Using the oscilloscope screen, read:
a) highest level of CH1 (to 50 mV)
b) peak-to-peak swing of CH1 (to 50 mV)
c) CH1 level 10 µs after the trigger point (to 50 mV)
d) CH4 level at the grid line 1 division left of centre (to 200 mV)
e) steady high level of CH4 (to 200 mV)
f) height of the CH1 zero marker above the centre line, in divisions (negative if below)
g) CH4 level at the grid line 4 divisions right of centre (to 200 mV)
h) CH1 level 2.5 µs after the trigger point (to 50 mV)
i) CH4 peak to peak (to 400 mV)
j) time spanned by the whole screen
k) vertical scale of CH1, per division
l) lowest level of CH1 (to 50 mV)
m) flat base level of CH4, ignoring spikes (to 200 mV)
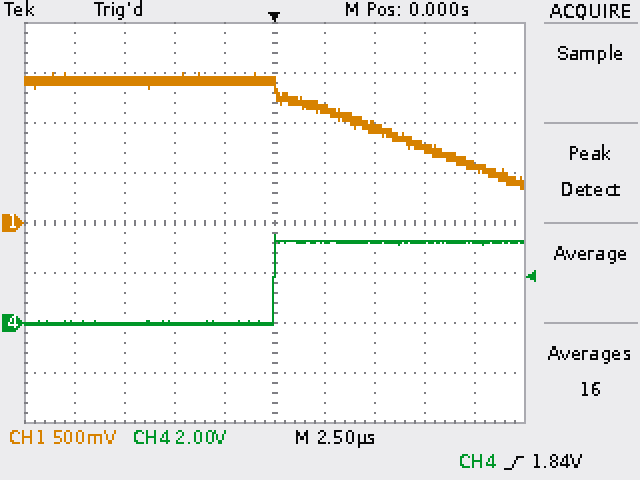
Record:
1.50 V
1.15 V
600 mV
0.0 V
3.2 V
0.0 div
3.2 V
1.15 V
3.6 V
25 µs
500 mV
350 mV
0.0 V
